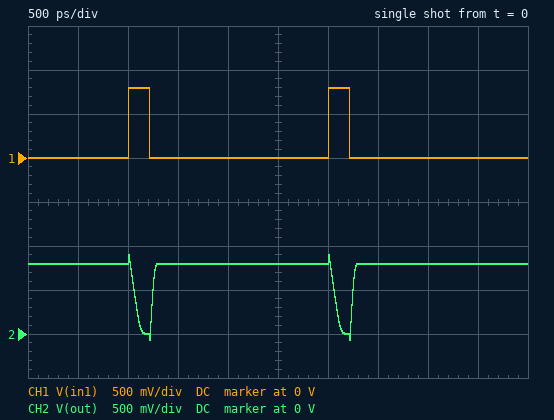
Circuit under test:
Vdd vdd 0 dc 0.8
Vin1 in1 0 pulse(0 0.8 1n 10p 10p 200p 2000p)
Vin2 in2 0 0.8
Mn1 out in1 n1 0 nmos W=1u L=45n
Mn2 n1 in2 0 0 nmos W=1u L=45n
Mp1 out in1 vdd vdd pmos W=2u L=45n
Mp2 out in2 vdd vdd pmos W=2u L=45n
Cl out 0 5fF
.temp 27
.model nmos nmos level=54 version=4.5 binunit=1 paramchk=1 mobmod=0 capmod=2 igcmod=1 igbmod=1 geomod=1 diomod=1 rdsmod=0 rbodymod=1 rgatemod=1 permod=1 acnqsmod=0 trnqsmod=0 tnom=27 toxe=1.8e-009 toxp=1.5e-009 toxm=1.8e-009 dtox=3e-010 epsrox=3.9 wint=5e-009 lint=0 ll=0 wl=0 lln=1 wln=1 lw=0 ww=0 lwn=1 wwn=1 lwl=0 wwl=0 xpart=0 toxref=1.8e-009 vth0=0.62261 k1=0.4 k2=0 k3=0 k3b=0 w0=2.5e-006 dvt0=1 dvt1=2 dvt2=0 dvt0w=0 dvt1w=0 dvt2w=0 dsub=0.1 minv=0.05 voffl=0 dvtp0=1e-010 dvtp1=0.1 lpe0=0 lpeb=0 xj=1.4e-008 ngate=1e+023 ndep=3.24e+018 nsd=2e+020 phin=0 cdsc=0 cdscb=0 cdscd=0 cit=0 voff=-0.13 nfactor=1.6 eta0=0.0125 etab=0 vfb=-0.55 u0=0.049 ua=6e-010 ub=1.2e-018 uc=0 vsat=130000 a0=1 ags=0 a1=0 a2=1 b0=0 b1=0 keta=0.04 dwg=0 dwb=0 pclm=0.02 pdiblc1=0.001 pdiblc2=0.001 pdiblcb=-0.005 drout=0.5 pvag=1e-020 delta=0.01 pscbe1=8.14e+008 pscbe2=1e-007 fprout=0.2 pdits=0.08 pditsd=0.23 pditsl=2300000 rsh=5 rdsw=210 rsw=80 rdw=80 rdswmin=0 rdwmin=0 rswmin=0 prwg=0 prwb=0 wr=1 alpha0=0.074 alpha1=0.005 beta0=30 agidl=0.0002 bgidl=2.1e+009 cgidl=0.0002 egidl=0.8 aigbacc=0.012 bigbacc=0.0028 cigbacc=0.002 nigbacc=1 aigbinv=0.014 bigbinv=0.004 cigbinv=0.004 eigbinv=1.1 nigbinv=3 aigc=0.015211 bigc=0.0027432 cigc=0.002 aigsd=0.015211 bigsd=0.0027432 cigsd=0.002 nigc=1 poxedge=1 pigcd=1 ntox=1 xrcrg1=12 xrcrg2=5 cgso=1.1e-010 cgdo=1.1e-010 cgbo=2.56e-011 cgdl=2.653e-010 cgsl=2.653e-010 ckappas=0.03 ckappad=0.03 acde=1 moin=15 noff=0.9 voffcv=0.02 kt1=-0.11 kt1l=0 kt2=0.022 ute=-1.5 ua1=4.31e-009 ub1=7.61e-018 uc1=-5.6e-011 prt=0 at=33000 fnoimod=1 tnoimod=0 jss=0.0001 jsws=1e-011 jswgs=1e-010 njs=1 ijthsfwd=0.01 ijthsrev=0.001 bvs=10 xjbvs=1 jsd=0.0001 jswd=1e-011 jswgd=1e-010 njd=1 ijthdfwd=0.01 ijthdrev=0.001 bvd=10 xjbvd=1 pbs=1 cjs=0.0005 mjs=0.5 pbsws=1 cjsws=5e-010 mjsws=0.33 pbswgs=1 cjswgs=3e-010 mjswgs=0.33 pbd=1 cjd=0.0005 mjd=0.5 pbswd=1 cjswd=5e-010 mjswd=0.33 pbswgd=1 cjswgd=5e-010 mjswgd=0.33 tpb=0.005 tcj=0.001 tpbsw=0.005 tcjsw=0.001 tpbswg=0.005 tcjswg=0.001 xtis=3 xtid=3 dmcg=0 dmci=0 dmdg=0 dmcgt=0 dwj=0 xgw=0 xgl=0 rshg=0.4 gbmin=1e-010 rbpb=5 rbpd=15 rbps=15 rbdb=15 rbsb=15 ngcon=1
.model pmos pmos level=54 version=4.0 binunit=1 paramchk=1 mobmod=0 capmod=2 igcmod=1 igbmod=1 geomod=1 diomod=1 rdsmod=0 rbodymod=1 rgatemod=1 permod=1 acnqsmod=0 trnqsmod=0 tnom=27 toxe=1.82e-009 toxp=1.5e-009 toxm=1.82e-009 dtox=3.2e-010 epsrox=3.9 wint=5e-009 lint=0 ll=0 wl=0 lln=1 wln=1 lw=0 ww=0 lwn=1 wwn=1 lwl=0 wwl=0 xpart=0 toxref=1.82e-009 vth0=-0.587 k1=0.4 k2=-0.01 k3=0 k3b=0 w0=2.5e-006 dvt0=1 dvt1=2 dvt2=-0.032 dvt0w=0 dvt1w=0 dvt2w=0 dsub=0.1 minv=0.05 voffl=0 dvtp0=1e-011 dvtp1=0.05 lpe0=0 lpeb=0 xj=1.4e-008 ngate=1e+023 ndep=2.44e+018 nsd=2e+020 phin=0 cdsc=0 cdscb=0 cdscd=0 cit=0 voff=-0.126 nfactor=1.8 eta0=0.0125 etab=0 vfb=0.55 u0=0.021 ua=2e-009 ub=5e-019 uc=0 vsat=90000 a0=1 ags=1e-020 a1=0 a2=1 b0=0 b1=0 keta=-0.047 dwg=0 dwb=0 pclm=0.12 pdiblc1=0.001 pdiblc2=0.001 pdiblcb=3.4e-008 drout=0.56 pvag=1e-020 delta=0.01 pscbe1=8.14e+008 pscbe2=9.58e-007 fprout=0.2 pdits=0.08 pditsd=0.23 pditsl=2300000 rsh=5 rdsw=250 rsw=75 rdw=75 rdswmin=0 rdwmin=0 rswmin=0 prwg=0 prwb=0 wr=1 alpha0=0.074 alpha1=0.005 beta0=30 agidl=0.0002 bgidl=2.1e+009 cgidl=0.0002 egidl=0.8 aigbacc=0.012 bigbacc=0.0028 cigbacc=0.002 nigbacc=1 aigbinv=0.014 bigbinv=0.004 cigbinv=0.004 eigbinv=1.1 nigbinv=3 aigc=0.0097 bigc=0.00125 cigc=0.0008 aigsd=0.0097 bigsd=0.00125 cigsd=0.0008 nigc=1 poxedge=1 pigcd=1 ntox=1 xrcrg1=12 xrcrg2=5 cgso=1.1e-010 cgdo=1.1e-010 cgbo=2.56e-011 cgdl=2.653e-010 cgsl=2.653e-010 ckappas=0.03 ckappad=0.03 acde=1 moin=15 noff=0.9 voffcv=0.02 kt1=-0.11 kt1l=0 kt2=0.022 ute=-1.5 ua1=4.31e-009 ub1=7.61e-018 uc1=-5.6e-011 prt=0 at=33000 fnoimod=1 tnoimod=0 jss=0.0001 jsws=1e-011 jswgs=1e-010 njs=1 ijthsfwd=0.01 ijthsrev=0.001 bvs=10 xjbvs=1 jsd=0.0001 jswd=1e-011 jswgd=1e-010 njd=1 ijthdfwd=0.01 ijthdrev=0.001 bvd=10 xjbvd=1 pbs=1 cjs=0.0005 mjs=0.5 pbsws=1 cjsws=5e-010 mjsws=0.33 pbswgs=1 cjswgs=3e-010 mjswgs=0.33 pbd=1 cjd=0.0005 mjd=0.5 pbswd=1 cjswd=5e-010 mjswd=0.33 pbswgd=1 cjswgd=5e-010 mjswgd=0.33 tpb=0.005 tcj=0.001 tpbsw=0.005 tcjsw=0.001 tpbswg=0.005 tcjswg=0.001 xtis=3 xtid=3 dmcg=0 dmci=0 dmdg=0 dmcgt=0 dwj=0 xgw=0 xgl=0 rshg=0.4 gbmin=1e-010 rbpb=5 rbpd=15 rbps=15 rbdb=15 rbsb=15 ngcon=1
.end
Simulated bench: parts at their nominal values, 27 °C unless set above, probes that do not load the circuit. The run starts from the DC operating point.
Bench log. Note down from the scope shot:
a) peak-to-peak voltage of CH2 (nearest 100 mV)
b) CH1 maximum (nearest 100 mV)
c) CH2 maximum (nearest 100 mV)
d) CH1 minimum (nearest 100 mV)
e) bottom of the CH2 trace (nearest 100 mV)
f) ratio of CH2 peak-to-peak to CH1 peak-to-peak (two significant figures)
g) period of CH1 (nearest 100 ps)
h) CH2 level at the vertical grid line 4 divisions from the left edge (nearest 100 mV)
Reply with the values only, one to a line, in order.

1.0 V
800 mV
900 mV
0 V
-100 mV
1.2
2.0 ns
800 mV
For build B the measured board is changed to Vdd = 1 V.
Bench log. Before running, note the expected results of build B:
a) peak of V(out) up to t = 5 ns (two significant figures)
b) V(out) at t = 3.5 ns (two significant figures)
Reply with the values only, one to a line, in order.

1.1 V
1.0 V
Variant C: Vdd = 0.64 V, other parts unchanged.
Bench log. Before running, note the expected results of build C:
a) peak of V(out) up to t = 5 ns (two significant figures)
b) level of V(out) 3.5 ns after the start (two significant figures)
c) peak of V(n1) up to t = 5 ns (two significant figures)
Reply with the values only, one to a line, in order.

740 mV
640 mV
78 mV
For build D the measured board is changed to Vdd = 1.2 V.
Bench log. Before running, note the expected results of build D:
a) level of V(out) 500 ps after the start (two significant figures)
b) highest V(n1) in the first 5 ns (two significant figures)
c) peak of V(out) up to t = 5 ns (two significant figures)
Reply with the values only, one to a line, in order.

1.2 V
97 mV
1.3 V
